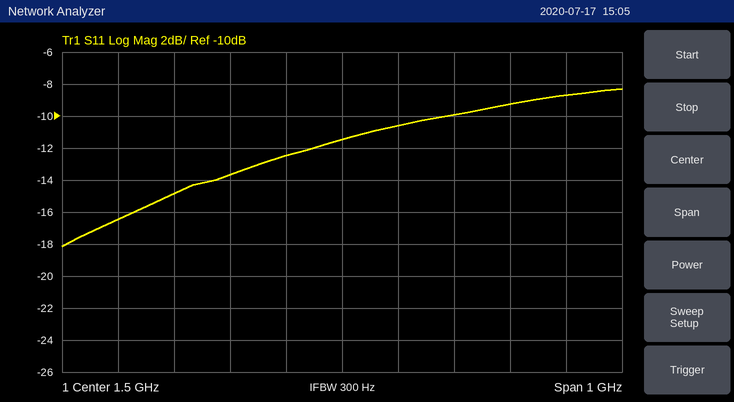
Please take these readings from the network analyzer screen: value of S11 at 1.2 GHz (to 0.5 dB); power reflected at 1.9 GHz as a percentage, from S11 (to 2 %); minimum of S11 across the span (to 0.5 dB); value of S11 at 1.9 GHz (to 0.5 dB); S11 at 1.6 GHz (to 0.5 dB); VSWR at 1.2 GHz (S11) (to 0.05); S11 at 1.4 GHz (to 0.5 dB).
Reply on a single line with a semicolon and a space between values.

-15.0 dB; 14 %; -18.0 dB; -8.5 dB; -10.5 dB; 1.45; -12.5 dB
